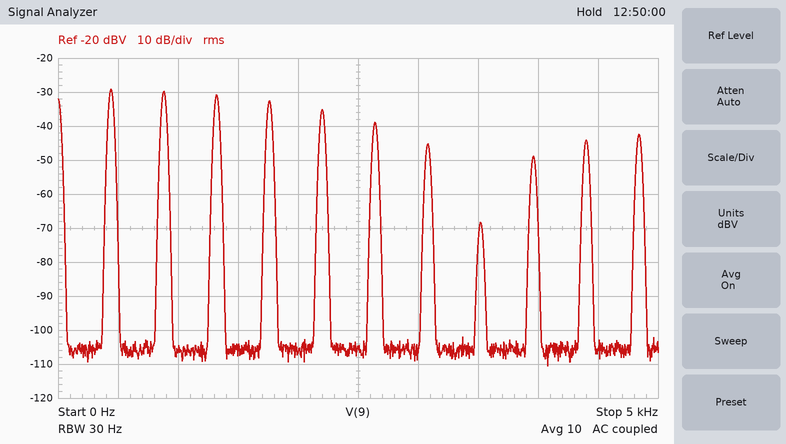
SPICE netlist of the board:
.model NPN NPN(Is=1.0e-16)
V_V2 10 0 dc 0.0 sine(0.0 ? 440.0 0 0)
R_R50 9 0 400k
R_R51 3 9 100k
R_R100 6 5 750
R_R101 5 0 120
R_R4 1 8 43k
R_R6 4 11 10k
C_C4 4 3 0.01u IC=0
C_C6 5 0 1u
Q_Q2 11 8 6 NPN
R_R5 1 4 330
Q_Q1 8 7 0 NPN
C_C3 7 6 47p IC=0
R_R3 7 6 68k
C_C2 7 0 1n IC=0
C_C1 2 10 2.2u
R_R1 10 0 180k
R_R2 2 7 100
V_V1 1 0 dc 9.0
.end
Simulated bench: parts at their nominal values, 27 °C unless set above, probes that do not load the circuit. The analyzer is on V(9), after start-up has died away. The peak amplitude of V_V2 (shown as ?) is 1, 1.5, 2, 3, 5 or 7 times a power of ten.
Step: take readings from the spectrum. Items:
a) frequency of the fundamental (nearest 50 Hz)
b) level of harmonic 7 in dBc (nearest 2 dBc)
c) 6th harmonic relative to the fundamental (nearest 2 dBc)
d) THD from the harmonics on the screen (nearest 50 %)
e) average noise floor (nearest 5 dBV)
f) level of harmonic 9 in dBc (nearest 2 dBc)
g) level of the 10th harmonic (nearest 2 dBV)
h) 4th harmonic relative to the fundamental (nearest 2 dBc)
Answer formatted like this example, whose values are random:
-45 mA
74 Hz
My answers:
450 Hz
-16 dBc
-10 dBc
150 %
-105 dBV
-20 dBc
-44 dBV
-4 dBc
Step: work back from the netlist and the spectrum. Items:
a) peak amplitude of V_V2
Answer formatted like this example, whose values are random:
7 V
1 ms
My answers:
150 mV
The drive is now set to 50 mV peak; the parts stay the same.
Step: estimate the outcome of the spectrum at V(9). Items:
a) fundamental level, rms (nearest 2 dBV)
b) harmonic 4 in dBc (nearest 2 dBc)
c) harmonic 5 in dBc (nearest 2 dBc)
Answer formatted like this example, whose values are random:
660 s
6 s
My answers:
-32 dBV
-2 dBc
-4 dBc
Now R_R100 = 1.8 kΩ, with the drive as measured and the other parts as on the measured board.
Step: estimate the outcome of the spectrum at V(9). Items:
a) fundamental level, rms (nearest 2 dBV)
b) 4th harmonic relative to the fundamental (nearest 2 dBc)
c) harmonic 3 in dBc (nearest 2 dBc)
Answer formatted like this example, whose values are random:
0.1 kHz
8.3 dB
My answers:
-26 dBV
-12 dBc
-6 dBc
